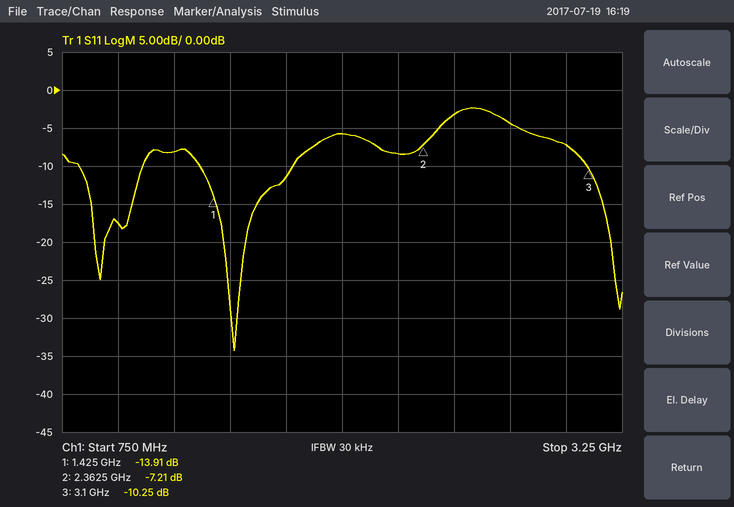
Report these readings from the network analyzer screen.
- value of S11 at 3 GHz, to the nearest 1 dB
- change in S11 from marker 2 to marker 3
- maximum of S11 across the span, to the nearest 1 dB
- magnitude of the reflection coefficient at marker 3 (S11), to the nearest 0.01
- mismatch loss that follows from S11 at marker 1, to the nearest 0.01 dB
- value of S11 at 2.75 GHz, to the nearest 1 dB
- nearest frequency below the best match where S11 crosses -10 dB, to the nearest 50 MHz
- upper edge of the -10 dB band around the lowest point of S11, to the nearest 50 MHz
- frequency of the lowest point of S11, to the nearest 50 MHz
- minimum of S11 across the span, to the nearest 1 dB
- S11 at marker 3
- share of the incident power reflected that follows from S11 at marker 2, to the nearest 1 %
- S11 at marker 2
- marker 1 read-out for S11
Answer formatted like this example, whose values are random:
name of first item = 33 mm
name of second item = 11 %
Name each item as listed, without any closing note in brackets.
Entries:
value of S11 at 3 GHz, to the nearest 1 dB = -7 dB
change in S11 from marker 2 to marker 3 = -3.04 dB
maximum of S11 across the span, to the nearest 1 dB = -2 dB
magnitude of the reflection coefficient at marker 3 (S11), to the nearest 0.01 = 0.31
mismatch loss that follows from S11 at marker 1, to the nearest 0.01 dB = 0.18 dB
value of S11 at 2.75 GHz, to the nearest 1 dB = -4 dB
nearest frequency below the best match where S11 crosses -10 dB, to the nearest 50 MHz = 1.35 GHz
upper edge of the -10 dB band around the lowest point of S11, to the nearest 50 MHz = 1.80 GHz
frequency of the lowest point of S11, to the nearest 50 MHz = 1.50 GHz
minimum of S11 across the span, to the nearest 1 dB = -34 dB
S11 at marker 3 = -10.25 dB
share of the incident power reflected that follows from S11 at marker 2, to the nearest 1 % = 19 %
S11 at marker 2 = -7.21 dB
marker 1 read-out for S11 = -13.91 dB
